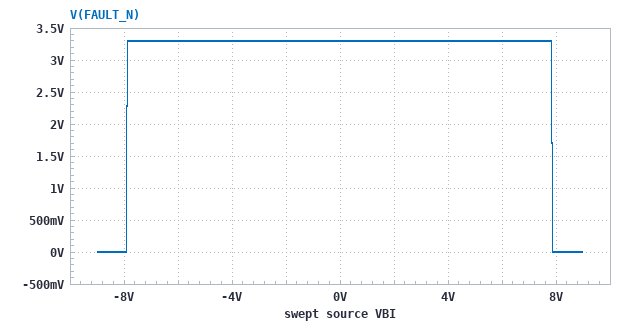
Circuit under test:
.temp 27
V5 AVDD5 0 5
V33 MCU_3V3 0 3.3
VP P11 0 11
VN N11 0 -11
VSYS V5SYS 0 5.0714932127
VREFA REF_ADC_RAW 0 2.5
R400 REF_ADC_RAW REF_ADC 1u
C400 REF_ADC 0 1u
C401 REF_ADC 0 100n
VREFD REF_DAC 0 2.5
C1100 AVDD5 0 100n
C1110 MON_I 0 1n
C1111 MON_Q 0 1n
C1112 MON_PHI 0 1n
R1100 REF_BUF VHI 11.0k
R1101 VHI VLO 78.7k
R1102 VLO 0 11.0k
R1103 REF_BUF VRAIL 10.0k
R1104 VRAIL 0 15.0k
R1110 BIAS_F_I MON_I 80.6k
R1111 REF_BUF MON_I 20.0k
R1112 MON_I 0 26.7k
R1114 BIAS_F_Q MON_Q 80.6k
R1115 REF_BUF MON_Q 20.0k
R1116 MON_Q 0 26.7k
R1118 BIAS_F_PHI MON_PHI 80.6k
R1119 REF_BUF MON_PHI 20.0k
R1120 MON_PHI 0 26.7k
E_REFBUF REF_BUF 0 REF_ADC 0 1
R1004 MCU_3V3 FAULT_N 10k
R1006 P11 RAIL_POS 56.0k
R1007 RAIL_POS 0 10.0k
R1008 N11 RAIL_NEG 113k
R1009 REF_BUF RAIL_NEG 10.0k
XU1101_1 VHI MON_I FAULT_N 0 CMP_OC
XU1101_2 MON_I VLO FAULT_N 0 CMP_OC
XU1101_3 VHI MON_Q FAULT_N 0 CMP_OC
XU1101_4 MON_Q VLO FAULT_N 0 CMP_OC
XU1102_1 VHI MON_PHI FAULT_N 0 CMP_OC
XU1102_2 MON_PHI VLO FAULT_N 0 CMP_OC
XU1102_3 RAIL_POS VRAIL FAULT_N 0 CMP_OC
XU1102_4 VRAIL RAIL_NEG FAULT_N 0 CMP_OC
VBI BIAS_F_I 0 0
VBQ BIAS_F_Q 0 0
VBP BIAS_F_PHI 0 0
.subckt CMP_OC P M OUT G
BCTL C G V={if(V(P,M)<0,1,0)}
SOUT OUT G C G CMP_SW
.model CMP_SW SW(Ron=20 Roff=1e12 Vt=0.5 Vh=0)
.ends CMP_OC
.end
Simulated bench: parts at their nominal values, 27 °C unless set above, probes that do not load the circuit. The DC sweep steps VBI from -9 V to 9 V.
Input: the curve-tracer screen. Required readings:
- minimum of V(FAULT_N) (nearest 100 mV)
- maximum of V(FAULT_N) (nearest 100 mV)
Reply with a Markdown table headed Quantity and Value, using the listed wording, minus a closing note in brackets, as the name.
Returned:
| Quantity | Value |
|---|---|
| minimum of V(FAULT_N) | 0 V |
| maximum of V(FAULT_N) | 3.3 V |
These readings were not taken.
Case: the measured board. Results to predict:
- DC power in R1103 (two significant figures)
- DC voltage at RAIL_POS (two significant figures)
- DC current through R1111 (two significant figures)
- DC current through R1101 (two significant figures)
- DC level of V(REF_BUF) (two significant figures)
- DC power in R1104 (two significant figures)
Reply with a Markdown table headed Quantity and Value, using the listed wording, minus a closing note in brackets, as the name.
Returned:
| Quantity | Value |
|---|---|
| DC power in R1103 | 100 µW |
| DC voltage at RAIL_POS | 1.7 V |
| DC current through R1111 | 62 µA |
| DC current through R1101 | 25 µA |
| DC level of V(REF_BUF) | 2.5 V |
| DC power in R1104 | 150 µW |
